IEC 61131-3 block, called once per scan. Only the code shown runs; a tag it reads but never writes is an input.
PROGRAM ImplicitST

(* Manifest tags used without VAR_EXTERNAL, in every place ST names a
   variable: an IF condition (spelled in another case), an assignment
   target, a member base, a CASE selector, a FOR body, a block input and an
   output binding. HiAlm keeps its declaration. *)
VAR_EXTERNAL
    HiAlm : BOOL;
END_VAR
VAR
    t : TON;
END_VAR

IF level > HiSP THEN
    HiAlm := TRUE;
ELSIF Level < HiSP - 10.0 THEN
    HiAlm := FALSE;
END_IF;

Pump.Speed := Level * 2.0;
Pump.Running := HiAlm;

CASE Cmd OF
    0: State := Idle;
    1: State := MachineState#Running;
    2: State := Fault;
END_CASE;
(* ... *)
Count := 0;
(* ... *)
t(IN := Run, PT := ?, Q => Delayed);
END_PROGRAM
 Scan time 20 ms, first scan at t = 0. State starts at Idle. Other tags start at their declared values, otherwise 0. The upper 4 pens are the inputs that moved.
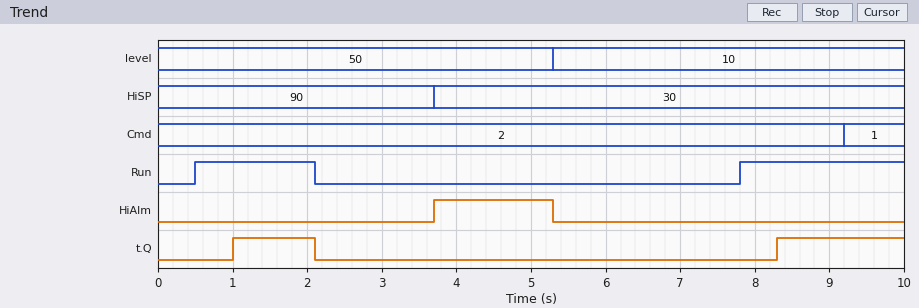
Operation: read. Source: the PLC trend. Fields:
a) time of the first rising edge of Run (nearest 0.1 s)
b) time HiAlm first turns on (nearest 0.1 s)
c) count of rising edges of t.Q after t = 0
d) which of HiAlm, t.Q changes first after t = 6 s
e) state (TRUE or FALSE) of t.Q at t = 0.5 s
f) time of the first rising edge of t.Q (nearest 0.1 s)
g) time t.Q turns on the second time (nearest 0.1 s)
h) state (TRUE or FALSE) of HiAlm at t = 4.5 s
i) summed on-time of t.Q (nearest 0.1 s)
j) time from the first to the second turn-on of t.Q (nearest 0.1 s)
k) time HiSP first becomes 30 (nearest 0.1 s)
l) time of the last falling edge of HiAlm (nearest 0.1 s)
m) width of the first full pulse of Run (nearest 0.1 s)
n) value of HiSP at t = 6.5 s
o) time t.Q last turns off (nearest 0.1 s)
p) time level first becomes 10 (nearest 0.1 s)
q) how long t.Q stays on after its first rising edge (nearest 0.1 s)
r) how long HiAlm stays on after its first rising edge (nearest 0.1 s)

0.5 s
3.7 s
2
t.Q
FALSE
1.0 s
8.3 s
TRUE
2.8 s
7.3 s
3.7 s
5.3 s
1.6 s
30
2.1 s
5.3 s
1.1 s
1.6 s
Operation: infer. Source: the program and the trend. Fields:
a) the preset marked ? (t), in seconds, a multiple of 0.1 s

0.5 s
